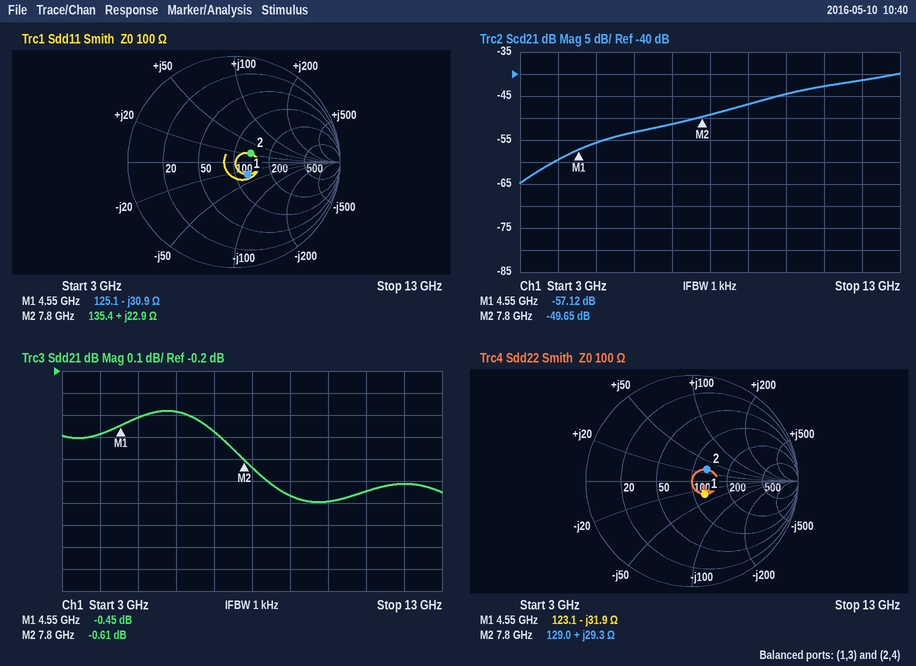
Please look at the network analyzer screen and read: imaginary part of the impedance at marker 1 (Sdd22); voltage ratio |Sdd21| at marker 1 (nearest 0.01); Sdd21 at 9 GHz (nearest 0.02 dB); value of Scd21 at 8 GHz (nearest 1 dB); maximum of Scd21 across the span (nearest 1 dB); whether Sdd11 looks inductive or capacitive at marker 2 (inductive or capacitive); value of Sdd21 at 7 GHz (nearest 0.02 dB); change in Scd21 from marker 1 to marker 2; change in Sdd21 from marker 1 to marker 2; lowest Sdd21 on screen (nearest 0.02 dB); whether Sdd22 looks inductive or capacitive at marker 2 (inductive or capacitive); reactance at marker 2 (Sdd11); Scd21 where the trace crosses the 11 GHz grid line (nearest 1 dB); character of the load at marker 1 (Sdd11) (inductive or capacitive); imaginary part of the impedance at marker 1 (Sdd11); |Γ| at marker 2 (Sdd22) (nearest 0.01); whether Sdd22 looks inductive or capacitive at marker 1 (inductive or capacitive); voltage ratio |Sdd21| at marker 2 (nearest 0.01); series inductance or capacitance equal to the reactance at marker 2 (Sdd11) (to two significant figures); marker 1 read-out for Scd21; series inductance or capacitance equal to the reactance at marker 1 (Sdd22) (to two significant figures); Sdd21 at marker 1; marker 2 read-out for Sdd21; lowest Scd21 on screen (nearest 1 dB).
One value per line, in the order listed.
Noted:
-31.9 Ω
0.95
-0.76 dB
-49 dB
-40 dB
inductive
-0.48 dB
7.47 dB
-0.16 dB
-0.80 dB
inductive
+22.9 Ω
-43 dB
capacitive
-30.9 Ω
0.18
capacitive
0.93
470 pH
-57.12 dB
1.1 pF
-0.45 dB
-0.61 dB
-65 dB
